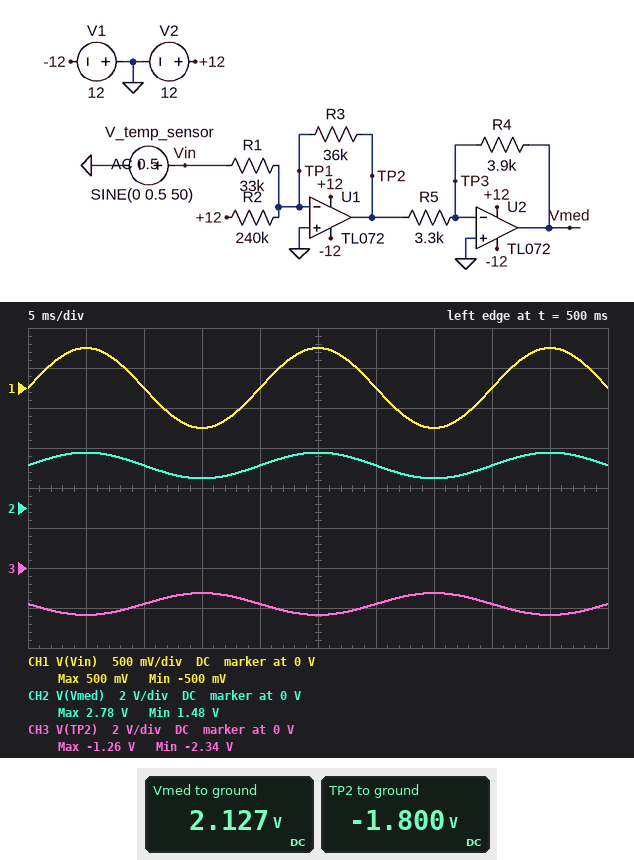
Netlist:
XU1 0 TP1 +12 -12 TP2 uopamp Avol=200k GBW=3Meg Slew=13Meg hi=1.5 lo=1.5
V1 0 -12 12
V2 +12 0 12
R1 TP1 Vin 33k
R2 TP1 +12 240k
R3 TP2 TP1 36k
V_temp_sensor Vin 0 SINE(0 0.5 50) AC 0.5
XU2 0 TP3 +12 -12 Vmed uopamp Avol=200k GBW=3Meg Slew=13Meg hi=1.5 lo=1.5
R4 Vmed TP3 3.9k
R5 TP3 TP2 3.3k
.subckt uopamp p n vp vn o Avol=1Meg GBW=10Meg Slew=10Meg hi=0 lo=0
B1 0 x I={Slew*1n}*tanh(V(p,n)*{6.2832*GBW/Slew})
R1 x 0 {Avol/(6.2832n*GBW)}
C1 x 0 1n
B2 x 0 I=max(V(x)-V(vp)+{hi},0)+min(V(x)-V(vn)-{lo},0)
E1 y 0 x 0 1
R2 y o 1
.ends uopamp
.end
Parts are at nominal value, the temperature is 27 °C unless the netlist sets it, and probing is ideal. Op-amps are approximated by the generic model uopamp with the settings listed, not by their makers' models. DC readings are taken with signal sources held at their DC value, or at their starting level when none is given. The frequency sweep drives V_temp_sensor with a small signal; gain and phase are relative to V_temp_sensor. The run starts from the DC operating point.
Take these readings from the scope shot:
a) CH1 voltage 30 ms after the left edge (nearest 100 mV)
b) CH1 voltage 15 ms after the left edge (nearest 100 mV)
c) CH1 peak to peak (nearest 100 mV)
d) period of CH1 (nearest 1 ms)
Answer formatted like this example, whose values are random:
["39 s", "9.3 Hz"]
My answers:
["0 V", "-500 mV", "1.0 V", "20 ms"]
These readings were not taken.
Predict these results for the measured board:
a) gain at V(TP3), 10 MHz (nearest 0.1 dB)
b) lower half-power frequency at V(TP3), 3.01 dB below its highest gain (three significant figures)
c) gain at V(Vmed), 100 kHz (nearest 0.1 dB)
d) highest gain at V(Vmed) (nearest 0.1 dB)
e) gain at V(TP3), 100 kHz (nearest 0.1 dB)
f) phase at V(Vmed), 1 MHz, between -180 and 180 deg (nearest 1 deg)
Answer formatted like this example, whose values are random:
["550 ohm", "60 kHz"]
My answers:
["-22.2 dB", "562 kHz", "2.2 dB", "2.2 dB", "-27.4 dB", "-73 deg"]
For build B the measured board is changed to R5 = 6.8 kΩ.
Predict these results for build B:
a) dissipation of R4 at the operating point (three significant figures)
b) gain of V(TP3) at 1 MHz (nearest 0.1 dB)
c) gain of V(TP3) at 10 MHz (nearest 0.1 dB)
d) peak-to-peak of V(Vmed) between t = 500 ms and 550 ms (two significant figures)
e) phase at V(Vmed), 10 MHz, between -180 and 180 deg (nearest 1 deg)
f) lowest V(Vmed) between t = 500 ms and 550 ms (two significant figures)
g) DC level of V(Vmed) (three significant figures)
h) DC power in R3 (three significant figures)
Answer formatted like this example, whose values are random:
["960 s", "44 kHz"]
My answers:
["273 µW", "-16.6 dB", "-25.7 dB", "630 mV", "-162 deg", "720 mV", "1.03 V", "90.0 µW"]
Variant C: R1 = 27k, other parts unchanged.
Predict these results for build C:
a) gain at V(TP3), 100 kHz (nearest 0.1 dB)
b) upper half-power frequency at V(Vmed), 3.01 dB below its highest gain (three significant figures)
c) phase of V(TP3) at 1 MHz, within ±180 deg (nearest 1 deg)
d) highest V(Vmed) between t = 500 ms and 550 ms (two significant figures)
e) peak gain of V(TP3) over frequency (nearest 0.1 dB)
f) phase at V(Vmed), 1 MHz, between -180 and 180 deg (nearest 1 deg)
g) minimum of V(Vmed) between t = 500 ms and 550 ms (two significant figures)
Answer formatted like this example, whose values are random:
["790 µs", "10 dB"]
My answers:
["-25.6 dB", "827 kHz", "-166 deg", "2.9 V", "-9.4 dB", "-76 deg", "1.3 V"]
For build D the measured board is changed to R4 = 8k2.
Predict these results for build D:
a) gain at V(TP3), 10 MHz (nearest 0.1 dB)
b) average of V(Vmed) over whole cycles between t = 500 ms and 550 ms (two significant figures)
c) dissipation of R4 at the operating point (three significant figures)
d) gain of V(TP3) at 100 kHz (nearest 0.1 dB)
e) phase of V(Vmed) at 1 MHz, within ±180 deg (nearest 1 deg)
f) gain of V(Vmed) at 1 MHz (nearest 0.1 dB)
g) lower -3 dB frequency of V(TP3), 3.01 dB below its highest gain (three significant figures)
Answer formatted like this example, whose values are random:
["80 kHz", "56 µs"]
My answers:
["-19.8 dB", "4.5 V", "2.44 mW", "-21.0 dB", "-86 deg", "3.0 dB", "437 kHz"]
